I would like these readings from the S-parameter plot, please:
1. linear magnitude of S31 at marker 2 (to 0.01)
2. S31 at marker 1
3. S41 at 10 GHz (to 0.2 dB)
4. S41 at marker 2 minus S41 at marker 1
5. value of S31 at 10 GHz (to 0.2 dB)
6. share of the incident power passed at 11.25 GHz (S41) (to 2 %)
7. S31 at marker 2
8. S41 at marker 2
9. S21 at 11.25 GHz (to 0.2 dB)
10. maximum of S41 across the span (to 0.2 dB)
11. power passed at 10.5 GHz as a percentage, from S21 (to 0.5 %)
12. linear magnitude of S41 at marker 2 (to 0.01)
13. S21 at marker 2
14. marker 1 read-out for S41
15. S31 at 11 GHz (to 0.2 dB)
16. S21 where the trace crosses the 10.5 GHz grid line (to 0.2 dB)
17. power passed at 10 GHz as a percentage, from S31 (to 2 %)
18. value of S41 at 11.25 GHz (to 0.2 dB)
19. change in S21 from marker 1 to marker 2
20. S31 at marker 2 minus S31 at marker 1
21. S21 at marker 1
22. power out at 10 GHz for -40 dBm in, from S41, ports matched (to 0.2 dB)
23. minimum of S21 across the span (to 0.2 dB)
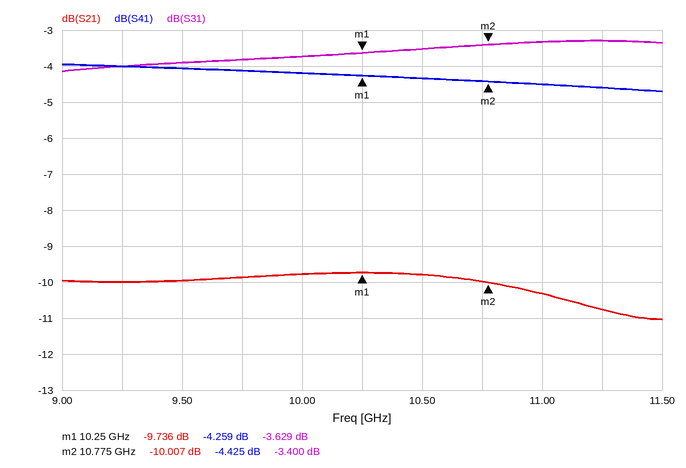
0.68
-3.629 dB
-4.2 dB
-0.166 dB
-3.8 dB
34 %
-3.400 dB
-4.425 dB
-10.8 dB
-4.0 dB
10.5 %
0.60
-10.007 dB
-4.259 dB
-3.4 dB
-9.8 dB
42 %
-4.6 dB
-0.271 dB
0.229 dB
-9.736 dB
-44.2 dBm
-11.0 dB
